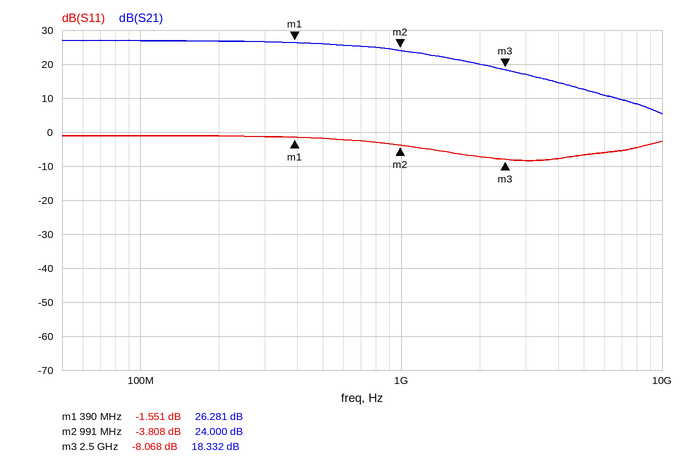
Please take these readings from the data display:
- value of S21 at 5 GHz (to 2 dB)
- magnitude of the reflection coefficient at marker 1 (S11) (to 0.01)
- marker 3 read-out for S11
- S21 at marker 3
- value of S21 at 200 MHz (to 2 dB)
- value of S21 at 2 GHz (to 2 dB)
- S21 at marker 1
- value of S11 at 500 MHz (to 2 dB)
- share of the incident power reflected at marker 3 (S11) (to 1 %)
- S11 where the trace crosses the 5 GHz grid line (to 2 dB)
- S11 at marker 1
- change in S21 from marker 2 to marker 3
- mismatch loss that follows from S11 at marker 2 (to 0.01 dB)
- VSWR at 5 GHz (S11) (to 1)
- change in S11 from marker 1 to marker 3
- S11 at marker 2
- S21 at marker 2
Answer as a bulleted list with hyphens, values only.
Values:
- 12 dB
- 0.84
- -8.068 dB
- 18.332 dB
- 26 dB
- 20 dB
- 26.281 dB
- -2 dB
- 16 %
- -6 dB
- -1.551 dB
- -5.668 dB
- 2.34 dB
- 3
- -6.517 dB
- -3.808 dB
- 24.000 dB
